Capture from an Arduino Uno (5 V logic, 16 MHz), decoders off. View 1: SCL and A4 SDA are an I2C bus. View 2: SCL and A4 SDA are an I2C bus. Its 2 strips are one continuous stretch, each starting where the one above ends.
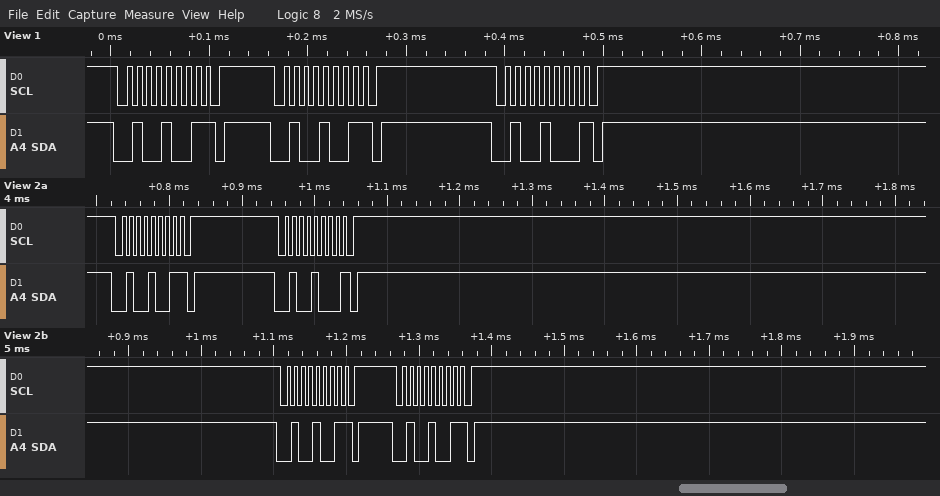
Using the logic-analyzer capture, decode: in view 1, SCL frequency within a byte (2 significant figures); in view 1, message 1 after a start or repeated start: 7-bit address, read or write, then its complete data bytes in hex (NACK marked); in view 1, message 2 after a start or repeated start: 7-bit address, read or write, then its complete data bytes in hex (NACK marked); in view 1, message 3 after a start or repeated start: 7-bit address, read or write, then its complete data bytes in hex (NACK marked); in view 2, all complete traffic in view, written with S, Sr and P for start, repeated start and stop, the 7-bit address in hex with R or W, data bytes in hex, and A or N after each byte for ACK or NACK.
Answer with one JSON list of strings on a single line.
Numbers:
["100 kHz", "0x24 read NACK", "0x24 read NACK", "0x24 write NACK", "S 24R N P S 24W N P S 24R N P S 24R N P"]
